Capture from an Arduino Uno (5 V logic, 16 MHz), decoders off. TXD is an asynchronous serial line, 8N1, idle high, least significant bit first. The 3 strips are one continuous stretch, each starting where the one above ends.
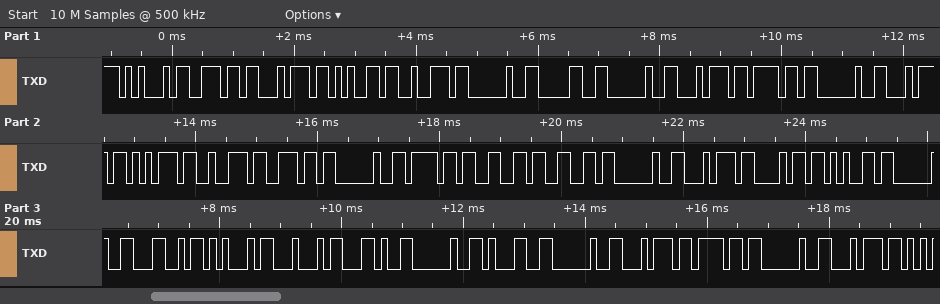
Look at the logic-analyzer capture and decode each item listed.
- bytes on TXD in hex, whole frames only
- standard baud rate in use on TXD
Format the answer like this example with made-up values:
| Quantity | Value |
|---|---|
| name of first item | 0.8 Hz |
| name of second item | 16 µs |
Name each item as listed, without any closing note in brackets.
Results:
| Quantity | Value |
|---|---|
| bytes on TXD in hex, whole frames only | 45 6E 74 65 72 20 30 20 74 6F 20 74 75 72 6E 20 6F 66 66 20 74 68 65 20 4C 45 44 2C 20 31 20 74 6F 20 74 |
| standard baud rate in use on TXD | 9600 baud |
